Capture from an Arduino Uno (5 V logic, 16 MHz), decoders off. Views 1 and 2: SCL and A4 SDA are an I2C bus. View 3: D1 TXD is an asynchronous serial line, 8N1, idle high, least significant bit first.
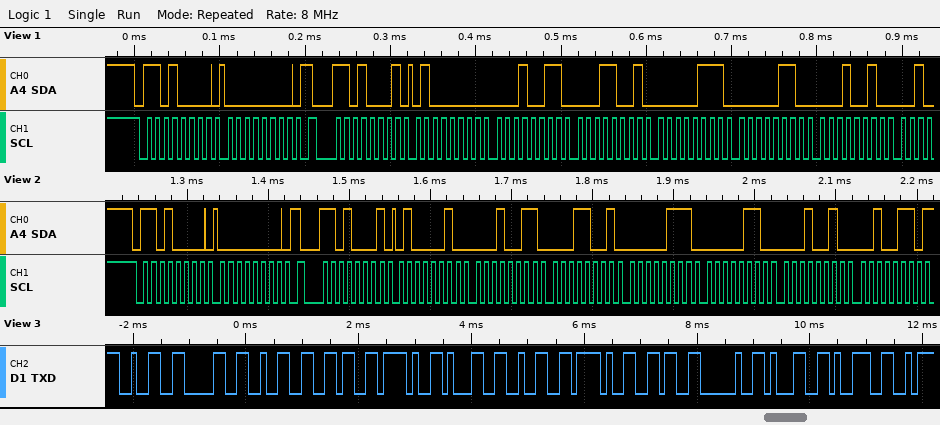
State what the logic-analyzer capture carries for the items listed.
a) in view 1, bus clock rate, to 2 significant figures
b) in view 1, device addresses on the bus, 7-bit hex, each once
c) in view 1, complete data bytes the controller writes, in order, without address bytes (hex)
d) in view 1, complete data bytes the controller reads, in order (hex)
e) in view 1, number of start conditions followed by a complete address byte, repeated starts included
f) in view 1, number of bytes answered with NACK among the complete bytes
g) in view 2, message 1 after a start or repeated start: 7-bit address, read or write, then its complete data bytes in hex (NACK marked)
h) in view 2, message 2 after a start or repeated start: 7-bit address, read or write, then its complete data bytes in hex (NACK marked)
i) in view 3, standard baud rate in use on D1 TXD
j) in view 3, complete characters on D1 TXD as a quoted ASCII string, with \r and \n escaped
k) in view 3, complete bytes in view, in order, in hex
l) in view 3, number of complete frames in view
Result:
100 kHz
0x68
00
40 13 19 07 06 12
2
0
0x68 write: 00
0x68 read: 42 13 19 07 06 12 26 NACK
9600 baud
"2026/12/6 19"
32 30 32 36 2F 31 32 2F 36 20 31 39
12
